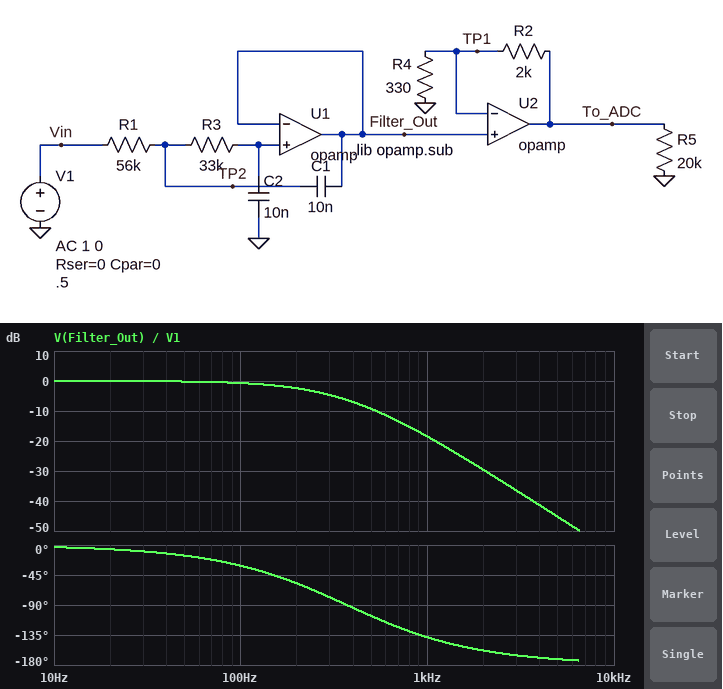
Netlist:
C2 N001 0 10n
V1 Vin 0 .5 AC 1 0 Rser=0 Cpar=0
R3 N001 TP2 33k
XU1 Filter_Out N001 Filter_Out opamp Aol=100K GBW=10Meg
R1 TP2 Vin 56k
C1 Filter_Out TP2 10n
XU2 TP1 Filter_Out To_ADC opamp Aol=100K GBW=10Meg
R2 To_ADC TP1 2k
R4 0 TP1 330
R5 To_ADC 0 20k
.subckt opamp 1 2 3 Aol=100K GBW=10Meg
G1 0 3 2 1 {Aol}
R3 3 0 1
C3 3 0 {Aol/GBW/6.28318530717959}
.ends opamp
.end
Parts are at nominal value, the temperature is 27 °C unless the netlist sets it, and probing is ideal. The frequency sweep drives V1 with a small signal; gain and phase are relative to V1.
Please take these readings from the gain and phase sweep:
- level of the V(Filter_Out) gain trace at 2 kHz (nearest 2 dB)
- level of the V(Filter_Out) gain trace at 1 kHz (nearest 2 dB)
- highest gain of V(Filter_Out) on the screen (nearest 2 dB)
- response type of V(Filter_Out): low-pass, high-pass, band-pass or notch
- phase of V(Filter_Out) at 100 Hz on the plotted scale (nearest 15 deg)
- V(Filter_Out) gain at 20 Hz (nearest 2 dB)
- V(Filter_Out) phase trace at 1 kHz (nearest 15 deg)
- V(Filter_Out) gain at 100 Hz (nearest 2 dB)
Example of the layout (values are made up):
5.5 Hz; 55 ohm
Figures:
-30 dB; -18 dB; 0 dB; low-pass; -30 deg; 0 dB; -135 deg; 0 dB
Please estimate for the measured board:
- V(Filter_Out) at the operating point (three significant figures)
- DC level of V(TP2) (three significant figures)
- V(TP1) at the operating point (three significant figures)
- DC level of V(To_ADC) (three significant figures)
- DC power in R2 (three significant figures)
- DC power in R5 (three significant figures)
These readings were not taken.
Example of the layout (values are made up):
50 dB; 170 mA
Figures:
500 mV; 500 mV; 500 mV; 3.53 V; 4.59 mW; 623 µW
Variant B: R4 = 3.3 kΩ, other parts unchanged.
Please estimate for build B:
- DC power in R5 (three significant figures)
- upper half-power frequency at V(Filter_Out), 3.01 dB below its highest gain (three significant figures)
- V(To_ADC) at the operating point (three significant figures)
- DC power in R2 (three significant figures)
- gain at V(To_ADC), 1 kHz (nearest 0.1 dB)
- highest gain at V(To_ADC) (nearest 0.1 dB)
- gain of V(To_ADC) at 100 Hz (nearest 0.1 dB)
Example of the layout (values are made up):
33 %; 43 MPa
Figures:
32.2 µW; 227 Hz; 803 mV; 45.9 µW; -14.4 dB; 4.1 dB; 3.4 dB
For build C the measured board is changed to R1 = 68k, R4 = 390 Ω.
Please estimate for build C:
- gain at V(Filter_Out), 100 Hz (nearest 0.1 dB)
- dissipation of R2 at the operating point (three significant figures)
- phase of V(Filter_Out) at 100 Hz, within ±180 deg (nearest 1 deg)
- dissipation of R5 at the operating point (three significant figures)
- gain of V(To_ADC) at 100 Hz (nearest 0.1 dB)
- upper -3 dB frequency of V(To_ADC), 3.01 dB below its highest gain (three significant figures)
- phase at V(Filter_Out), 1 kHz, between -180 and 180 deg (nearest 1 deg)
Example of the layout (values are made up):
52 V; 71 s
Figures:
-0.9 dB; 3.29 mW; -35 deg; 469 µW; 14.8 dB; 198 Hz; -141 deg
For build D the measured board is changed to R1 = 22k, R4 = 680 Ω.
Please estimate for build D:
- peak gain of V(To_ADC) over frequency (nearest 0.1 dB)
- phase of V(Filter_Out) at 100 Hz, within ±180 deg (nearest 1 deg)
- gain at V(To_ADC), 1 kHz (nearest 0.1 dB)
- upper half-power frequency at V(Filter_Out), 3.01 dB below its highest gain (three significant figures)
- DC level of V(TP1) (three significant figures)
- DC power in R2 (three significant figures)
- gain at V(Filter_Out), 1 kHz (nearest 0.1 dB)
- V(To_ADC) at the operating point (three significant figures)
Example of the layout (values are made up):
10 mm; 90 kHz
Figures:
11.9 dB; -20 deg; 0 dB; 369 Hz; 500 mV; 1.08 mW; -11.9 dB; 1.97 V
